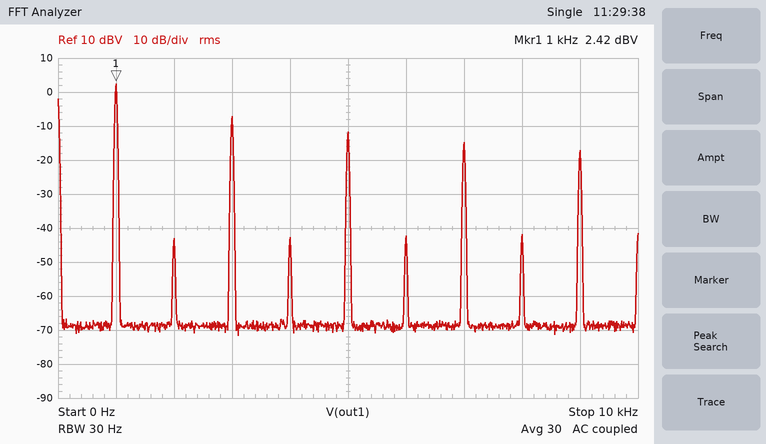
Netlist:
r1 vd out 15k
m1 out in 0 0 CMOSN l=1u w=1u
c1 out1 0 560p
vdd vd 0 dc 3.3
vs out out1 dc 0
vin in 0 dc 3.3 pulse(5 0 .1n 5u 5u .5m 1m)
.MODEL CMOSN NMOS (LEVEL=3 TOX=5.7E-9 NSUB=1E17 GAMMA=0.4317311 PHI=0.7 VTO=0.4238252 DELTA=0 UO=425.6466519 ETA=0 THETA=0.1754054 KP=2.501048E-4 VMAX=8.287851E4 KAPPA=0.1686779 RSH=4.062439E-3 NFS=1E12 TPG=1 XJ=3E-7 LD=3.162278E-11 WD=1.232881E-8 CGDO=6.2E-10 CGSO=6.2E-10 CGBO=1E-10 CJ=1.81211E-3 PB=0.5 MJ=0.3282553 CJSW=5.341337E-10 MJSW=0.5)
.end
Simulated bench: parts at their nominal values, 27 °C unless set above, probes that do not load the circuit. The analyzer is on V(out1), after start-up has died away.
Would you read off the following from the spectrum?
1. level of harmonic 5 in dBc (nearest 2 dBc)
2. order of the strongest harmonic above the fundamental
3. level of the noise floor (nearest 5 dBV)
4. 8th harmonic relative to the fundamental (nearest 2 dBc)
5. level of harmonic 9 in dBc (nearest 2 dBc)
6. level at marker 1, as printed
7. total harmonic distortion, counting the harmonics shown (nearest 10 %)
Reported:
-14 dBc
3
-70 dBV
-44 dBc
-20 dBc
2.42 dBV
40 %
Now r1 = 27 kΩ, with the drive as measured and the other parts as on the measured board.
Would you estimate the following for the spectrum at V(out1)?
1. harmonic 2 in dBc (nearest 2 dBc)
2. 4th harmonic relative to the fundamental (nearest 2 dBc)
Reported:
-32 dBc
-32 dBc
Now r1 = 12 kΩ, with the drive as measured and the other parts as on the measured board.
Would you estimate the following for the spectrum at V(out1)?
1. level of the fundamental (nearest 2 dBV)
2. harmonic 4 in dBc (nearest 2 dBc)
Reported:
2 dBV
-56 dBc
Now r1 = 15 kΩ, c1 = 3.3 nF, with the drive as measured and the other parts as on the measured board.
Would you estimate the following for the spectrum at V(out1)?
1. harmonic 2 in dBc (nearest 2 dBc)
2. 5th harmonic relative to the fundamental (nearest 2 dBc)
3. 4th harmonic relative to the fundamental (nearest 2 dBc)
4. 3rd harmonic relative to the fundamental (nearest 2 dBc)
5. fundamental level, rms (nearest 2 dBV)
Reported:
-20 dBc
-16 dBc
-24 dBc
-10 dBc
2 dBV
